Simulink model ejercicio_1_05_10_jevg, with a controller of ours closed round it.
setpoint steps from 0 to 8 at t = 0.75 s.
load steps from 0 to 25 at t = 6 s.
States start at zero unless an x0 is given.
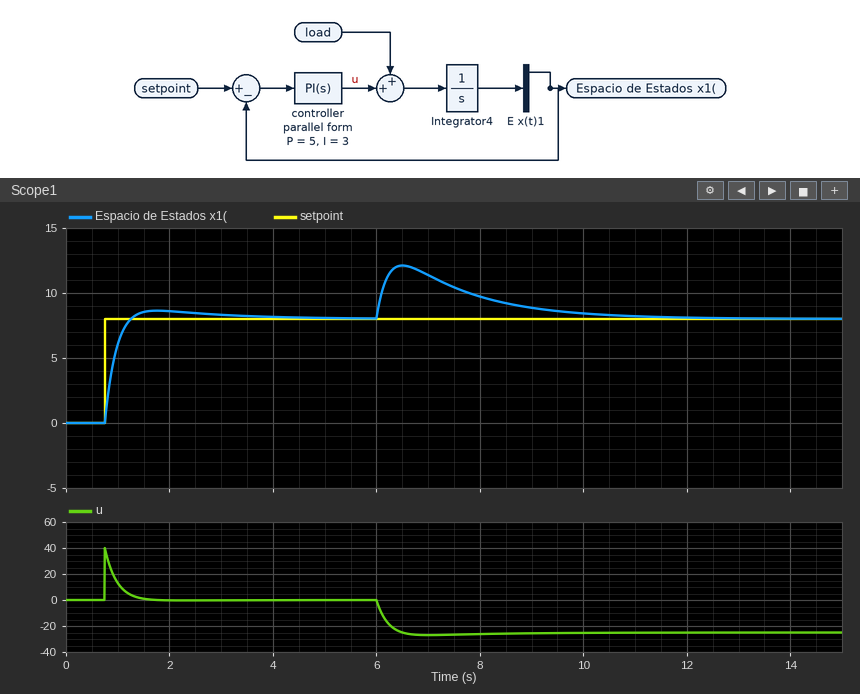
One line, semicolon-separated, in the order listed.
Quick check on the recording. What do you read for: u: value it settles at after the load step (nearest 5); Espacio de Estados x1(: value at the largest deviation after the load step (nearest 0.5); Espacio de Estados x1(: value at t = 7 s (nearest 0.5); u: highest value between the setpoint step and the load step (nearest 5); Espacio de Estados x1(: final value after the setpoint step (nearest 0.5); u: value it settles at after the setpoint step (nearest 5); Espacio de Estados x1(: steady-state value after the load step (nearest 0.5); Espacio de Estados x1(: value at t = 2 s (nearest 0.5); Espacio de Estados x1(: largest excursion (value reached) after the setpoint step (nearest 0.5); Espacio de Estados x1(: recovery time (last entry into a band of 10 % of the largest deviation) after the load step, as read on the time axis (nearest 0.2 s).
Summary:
-25; 12.0; 11.5; 40; 8.0; 0; 8.0; 8.5; 8.5; 10.0 s
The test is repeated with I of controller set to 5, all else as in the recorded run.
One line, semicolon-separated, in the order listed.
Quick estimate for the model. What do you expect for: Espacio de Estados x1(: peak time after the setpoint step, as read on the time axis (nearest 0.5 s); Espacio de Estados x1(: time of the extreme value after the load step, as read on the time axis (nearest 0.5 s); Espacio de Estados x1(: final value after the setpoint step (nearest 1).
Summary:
1.5 s; 6.5 s; 8
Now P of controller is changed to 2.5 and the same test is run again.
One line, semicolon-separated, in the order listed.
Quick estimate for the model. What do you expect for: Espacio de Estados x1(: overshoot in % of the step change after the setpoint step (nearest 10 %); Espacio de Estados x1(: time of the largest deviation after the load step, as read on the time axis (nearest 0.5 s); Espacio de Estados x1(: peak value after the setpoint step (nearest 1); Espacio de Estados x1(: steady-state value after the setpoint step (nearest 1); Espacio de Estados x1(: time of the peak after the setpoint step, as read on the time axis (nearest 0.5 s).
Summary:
20 %; 6.5 s; 10; 8; 2.0 s
